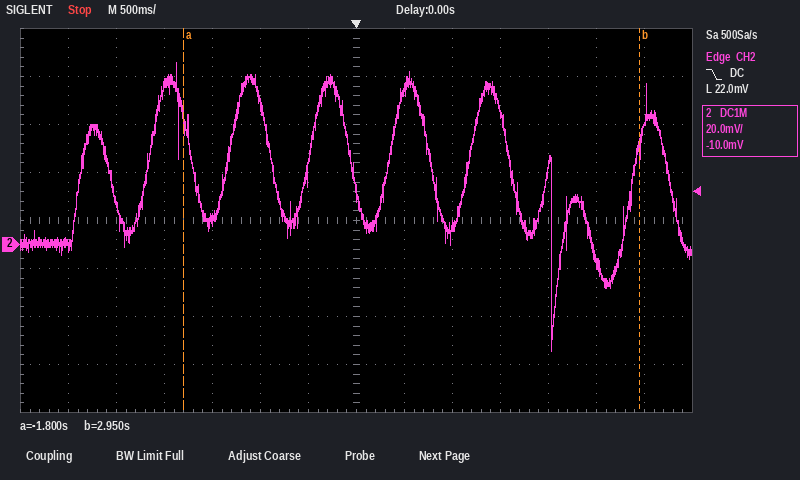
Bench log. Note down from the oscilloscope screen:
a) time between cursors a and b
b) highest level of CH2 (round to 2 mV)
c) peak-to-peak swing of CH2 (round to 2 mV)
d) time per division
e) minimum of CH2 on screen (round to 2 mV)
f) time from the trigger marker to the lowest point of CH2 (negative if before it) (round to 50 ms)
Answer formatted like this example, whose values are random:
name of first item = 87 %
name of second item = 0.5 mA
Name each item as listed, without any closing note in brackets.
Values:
time between cursors a and b = 4.75 s
highest level of CH2 = 76 mV
peak-to-peak swing of CH2 = 120 mV
time per division = 500 ms
minimum of CH2 on screen = -44 mV
time from the trigger marker to the lowest point of CH2 (negative if before it) = +2.05 s
